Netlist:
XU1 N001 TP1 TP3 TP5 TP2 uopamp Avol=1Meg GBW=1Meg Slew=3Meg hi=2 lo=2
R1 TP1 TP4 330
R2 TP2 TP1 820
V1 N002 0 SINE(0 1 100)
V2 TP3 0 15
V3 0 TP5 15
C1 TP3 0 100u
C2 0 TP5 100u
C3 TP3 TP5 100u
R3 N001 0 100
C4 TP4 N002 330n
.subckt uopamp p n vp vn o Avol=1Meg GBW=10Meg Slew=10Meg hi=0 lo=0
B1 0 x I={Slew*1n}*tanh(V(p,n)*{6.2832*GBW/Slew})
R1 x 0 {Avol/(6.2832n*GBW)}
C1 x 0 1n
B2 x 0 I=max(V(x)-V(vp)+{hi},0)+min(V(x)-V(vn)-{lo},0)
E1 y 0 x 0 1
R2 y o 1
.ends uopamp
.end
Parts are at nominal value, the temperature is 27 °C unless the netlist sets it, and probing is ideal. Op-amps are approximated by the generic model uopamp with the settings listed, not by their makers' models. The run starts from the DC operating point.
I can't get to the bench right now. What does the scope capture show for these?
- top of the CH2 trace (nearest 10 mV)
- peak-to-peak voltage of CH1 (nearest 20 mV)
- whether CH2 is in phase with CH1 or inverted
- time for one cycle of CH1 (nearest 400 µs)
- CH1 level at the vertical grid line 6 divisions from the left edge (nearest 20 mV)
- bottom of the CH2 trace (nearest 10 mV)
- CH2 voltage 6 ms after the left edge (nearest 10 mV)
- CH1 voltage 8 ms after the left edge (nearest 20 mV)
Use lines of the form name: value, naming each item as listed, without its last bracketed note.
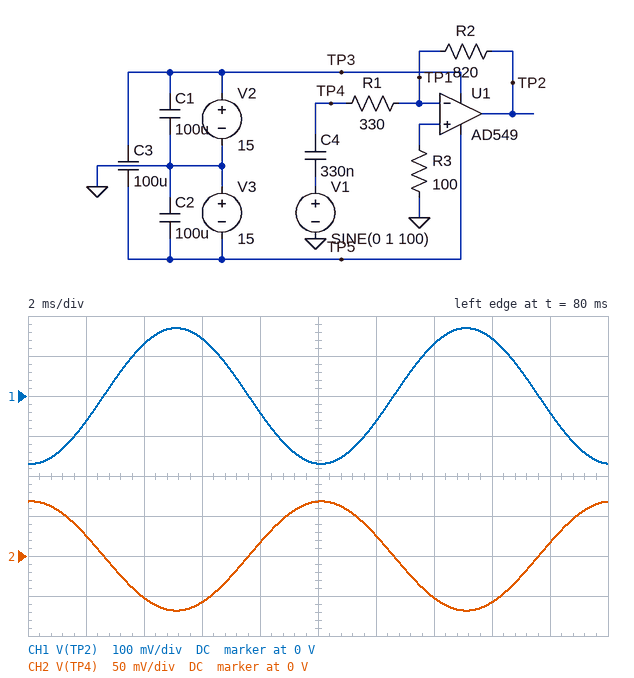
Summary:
top of the CH2 trace: 70 mV
peak-to-peak voltage of CH1: 340 mV
whether CH2 is in phase with CH1 or inverted: inverted
time for one cycle of CH1: 10.0 ms
CH1 level at the vertical grid line 6 divisions from the left edge: -60 mV
bottom of the CH2 trace: -70 mV
CH2 voltage 6 ms after the left edge: -60 mV
CH1 voltage 8 ms after the left edge: -40 mV
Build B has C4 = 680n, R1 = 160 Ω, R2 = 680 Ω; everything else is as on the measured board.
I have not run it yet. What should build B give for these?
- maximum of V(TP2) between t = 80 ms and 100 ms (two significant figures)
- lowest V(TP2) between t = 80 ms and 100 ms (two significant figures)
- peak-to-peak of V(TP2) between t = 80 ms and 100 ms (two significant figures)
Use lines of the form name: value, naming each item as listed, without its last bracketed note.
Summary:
maximum of V(TP2) between t = 80 ms and 100 ms: 290 mV
lowest V(TP2) between t = 80 ms and 100 ms: -290 mV
peak-to-peak of V(TP2) between t = 80 ms and 100 ms: 580 mV
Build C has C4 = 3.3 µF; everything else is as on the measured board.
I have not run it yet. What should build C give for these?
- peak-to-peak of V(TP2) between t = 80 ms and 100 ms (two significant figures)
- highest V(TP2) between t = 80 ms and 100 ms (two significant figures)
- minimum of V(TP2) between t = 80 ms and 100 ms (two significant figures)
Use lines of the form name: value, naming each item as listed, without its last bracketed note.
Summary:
peak-to-peak of V(TP2) between t = 80 ms and 100 ms: 2.8 V
highest V(TP2) between t = 80 ms and 100 ms: 1.4 V
minimum of V(TP2) between t = 80 ms and 100 ms: -1.4 V
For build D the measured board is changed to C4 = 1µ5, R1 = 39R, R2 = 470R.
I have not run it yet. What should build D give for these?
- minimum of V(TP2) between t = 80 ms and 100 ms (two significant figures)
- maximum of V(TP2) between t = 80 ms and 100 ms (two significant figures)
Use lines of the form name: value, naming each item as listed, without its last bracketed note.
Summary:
minimum of V(TP2) between t = 80 ms and 100 ms: -440 mV
maximum of V(TP2) between t = 80 ms and 100 ms: 440 mV
